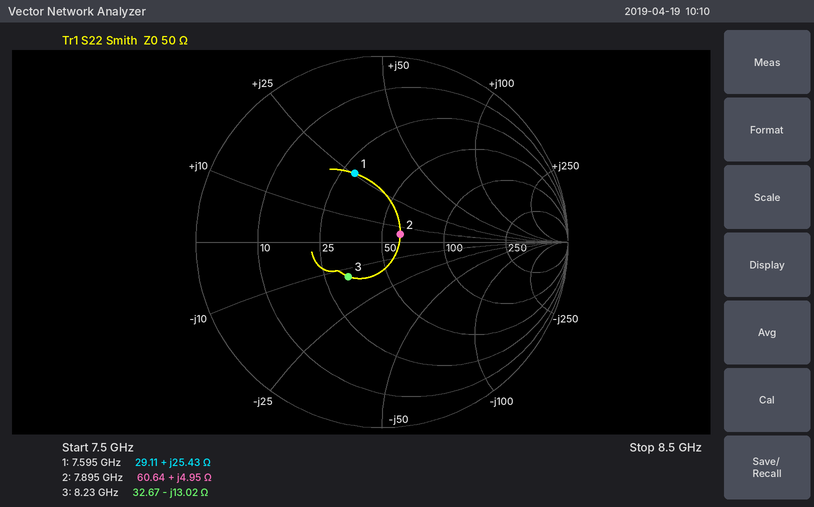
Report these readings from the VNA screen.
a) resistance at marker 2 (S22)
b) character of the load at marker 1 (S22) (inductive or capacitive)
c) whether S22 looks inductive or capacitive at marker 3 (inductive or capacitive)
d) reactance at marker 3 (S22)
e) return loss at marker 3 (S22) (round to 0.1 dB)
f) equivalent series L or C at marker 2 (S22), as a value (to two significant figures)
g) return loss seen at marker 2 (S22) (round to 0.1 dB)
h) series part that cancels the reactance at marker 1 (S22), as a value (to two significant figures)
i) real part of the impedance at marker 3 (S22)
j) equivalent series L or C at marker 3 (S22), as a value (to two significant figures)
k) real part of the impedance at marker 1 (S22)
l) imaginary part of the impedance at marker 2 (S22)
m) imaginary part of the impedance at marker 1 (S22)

60.64 Ω
inductive
capacitive
-13.02 Ω
11.7 dB
100 pH
19.5 dB
820 fF
32.67 Ω
1.5 pF
29.11 Ω
+4.95 Ω
+25.43 Ω
